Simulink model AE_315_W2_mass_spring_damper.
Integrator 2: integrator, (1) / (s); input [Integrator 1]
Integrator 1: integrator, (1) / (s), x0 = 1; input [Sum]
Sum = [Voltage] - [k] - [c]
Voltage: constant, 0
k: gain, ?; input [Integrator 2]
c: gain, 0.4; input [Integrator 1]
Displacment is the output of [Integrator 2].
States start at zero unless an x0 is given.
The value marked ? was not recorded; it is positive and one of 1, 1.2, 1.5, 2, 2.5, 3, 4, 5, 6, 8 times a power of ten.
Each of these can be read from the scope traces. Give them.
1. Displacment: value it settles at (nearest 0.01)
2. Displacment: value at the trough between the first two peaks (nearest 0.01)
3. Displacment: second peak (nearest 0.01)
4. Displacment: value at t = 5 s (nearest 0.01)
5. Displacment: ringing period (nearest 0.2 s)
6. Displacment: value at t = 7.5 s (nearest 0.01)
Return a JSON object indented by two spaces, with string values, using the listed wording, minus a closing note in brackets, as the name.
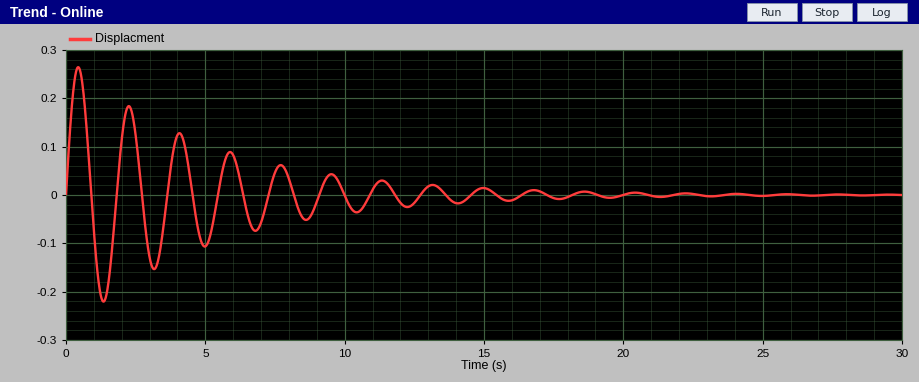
{
  "Displacment: value it settles at": "0.00",
  "Displacment: value at the trough between the first two peaks": "-0.22",
  "Displacment: second peak": "0.18",
  "Displacment: value at t = 5 s": "-0.11",
  "Displacment: ringing period": "1.8 s",
  "Displacment: value at t = 7.5 s": "0.05"
}
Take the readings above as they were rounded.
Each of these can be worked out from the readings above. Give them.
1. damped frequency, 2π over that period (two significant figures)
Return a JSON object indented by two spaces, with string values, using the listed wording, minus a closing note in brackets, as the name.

{
  "damped frequency, 2π over that period": "3.5 rad/s"
}
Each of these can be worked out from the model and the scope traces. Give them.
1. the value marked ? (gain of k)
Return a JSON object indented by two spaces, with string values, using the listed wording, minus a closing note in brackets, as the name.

{
  "the value marked ?": "12"
}
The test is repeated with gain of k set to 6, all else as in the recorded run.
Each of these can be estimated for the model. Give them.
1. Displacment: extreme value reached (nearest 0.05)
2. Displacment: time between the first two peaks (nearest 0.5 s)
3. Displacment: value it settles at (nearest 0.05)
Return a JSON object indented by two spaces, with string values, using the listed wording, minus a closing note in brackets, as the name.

{
  "Displacment: extreme value reached": "0.35",
  "Displacment: time between the first two peaks": "2.5 s",
  "Displacment: value it settles at": "0.00"
}
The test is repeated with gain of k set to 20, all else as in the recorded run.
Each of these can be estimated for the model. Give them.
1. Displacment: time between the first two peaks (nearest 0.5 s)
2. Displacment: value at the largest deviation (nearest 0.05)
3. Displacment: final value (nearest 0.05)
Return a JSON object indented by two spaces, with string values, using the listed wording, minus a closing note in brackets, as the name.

{
  "Displacment: time between the first two peaks": "1.5 s",
  "Displacment: value at the largest deviation": "0.20",
  "Displacment: final value": "0.00"
}
